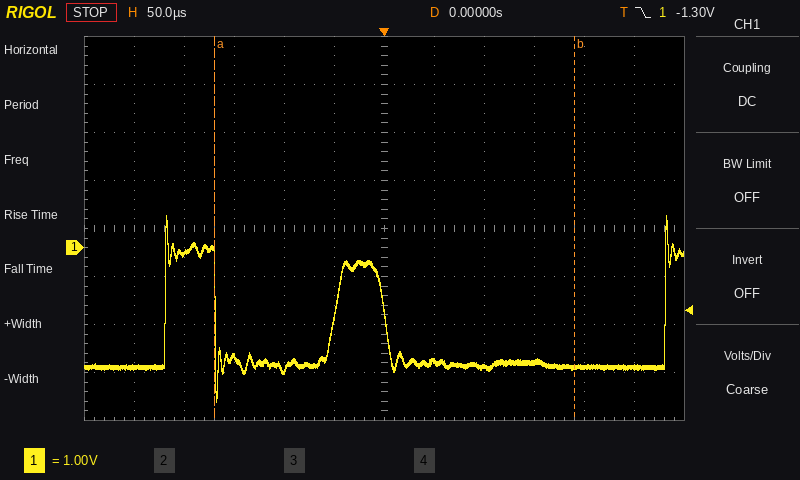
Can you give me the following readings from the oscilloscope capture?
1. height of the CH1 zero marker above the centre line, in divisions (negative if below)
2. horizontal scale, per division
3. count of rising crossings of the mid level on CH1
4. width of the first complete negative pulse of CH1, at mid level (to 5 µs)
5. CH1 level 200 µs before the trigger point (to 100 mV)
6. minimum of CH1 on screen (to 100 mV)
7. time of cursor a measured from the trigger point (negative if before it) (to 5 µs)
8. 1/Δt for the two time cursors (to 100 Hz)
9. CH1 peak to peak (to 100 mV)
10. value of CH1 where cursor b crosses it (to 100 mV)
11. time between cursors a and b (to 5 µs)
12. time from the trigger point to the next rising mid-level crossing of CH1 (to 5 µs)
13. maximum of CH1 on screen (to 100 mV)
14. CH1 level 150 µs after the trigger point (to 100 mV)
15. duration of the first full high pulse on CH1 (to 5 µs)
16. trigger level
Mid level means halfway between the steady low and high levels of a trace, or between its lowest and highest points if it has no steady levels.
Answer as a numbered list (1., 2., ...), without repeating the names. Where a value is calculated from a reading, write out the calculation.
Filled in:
1. -0.4 div
2. 50 µs
3. 3
4. 120 µs
5. -100 mV
6. -3.2 V
7. -170 µs
8. 1 / 360 µs ≈ 2.8 kHz
9. 700 mV − (-3.2 V) = 3.9 V
10. -2.5 V
11. 360 µs
12. 280 µs
13. 700 mV
14. -2.4 V
15. 50 µs
16. -1.30 V
